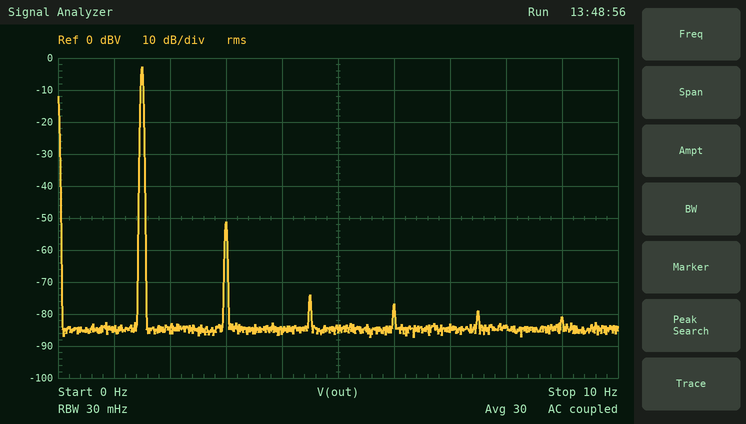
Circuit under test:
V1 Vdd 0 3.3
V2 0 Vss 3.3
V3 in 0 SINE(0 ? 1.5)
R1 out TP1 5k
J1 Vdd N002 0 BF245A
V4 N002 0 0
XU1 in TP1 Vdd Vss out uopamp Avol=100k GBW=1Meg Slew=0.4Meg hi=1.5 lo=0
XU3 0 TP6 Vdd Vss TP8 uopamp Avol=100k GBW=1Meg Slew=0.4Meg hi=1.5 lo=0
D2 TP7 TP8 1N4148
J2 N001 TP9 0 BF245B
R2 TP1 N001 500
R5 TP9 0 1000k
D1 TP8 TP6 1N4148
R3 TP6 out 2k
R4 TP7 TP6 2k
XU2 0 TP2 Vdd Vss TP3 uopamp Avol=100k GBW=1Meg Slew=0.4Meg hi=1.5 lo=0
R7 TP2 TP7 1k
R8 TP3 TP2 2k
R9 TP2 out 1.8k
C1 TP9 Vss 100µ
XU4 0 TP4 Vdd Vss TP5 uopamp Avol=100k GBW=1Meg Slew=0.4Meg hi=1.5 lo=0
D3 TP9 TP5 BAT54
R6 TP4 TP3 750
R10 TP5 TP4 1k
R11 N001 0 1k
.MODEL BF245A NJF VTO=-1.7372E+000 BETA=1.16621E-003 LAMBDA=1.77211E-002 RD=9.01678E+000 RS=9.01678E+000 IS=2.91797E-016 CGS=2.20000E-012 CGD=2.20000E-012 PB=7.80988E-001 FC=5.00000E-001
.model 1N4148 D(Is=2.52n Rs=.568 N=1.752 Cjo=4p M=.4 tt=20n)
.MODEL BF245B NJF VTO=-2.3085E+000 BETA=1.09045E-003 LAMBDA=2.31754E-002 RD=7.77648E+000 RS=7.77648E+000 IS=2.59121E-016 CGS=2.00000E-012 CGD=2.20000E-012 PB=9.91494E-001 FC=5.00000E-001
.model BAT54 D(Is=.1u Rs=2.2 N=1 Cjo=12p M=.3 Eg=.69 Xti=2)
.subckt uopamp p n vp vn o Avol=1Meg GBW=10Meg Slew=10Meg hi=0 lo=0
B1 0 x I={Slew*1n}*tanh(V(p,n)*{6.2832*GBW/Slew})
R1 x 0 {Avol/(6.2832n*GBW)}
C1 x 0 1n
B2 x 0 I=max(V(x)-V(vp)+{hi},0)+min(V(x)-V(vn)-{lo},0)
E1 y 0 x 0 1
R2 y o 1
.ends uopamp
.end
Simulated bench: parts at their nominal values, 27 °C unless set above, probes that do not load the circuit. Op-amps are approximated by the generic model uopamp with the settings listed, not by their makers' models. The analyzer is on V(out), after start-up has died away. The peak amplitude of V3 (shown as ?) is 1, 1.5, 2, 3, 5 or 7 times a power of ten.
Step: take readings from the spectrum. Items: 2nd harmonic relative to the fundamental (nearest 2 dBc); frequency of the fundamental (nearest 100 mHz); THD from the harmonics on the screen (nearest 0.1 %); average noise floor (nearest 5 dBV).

-48 dBc
1.5 Hz
0.4 %
-85 dBV
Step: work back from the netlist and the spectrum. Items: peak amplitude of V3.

150 mV
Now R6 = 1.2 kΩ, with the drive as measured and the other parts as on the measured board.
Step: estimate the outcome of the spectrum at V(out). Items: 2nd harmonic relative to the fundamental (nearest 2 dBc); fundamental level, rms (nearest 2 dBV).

-54 dBc
-2 dBV
